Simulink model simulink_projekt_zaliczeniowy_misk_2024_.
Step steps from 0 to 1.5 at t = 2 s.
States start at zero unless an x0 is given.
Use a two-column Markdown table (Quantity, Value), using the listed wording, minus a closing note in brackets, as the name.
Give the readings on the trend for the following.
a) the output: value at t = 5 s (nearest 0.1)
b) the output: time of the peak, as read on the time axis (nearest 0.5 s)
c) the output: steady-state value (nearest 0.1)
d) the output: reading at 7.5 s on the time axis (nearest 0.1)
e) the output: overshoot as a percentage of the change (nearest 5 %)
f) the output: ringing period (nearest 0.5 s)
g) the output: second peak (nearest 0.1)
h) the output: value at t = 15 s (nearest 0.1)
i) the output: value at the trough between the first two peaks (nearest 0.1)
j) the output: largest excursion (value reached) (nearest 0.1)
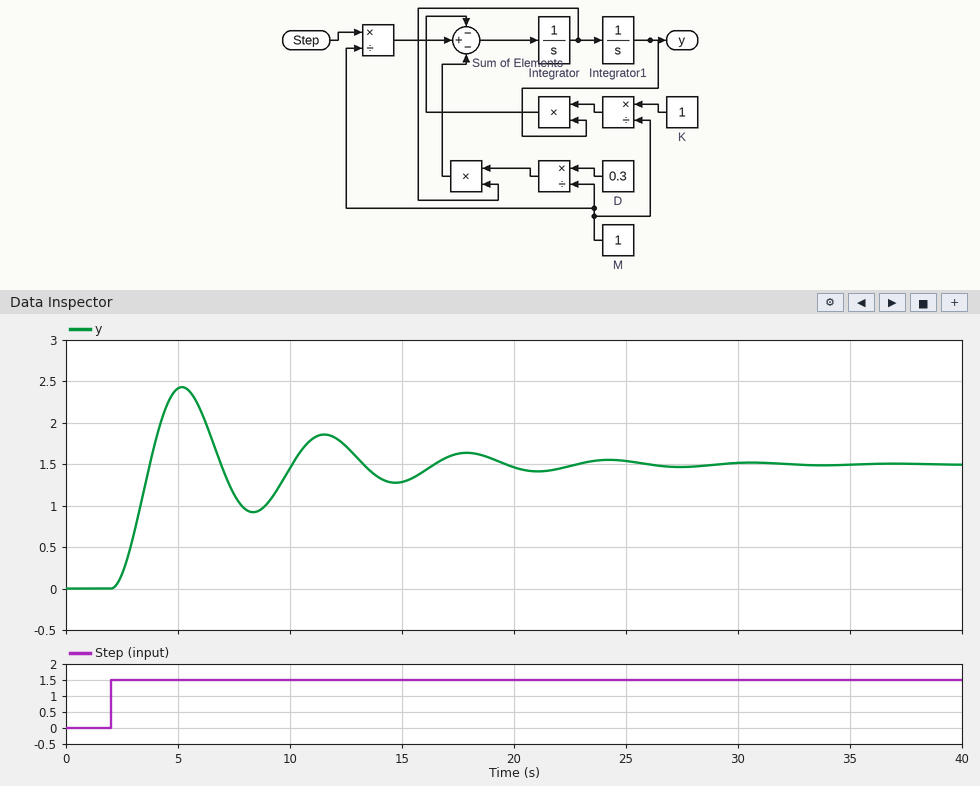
| Quantity | Value |
|---|---|
| the output: value at t = 5 s | 2.4 |
| the output: time of the peak, as read on the time axis | 5.0 s |
| the output: steady-state value | 1.5 |
| the output: reading at 7.5 s on the time axis | 1.1 |
| the output: overshoot as a percentage of the change | 60 % |
| the output: ringing period | 6.5 s |
| the output: second peak | 1.9 |
| the output: value at t = 15 s | 1.3 |
| the output: value at the trough between the first two peaks | 0.9 |
| the output: largest excursion (value reached) | 2.4 |
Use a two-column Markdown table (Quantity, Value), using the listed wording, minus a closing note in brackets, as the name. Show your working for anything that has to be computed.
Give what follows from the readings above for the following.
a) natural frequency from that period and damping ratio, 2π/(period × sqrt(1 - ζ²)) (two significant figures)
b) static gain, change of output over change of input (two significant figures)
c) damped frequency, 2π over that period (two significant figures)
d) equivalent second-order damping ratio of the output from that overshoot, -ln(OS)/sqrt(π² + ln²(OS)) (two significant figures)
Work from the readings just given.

| Quantity | Value |
|---|---|
| natural frequency from that period and damping ratio, 2π/(period × sqrt(1 - ζ²)) | 2π / (6.5 × sqrt(1 - 0.16²)) = 0.98 rad/s |
| static gain, change of output over change of input | (1.5 - 0) / (1.5 - 0) = 1.0 |
| damped frequency, 2π over that period | 2π / 6.5 = 0.97 rad/s |
| equivalent second-order damping ratio of the output from that overshoot, -ln(OS)/sqrt(π² + ln²(OS)) | ln(0.6) = -0.511; 0.511 / sqrt(9.870 + 0.261) = 0.16 |
